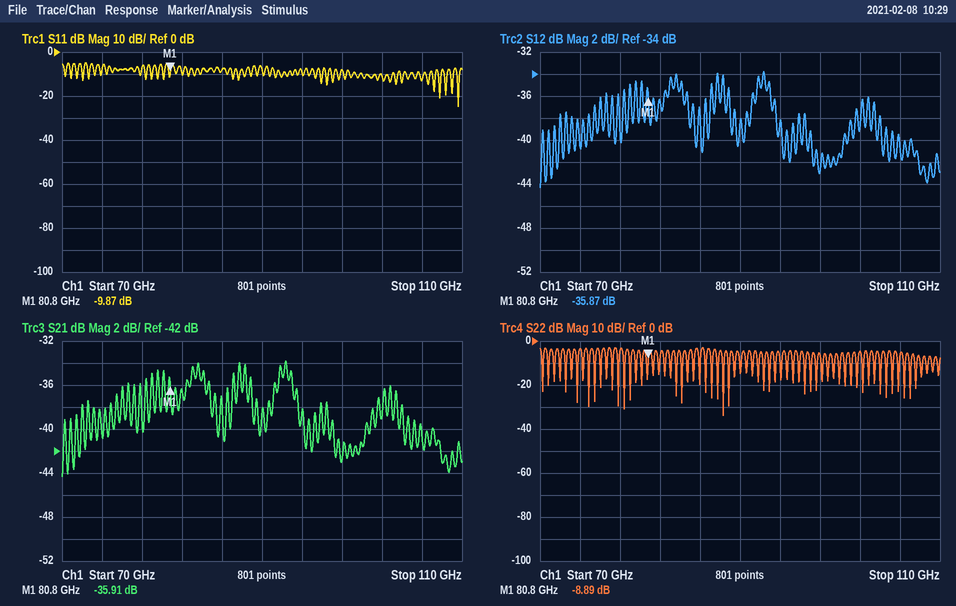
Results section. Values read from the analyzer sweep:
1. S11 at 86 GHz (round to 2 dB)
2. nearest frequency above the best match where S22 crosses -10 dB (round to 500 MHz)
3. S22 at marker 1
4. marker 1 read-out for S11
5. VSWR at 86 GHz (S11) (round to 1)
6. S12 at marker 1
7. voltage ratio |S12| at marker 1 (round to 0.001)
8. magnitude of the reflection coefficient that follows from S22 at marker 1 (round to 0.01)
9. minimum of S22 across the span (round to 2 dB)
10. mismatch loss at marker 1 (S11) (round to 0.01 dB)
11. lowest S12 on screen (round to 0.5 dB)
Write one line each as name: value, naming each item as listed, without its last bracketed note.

S11 at 86 GHz: -8 dB
nearest frequency above the best match where S22 crosses -10 dB: 88.5 GHz
S22 at marker 1: -8.89 dB
marker 1 read-out for S11: -9.87 dB
VSWR at 86 GHz (S11): 2
S12 at marker 1: -35.87 dB
voltage ratio |S12| at marker 1: 0.016
magnitude of the reflection coefficient that follows from S22 at marker 1: 0.36
minimum of S22 across the span: -34 dB
mismatch loss at marker 1 (S11): 0.47 dB
lowest S12 on screen: -44.5 dB
